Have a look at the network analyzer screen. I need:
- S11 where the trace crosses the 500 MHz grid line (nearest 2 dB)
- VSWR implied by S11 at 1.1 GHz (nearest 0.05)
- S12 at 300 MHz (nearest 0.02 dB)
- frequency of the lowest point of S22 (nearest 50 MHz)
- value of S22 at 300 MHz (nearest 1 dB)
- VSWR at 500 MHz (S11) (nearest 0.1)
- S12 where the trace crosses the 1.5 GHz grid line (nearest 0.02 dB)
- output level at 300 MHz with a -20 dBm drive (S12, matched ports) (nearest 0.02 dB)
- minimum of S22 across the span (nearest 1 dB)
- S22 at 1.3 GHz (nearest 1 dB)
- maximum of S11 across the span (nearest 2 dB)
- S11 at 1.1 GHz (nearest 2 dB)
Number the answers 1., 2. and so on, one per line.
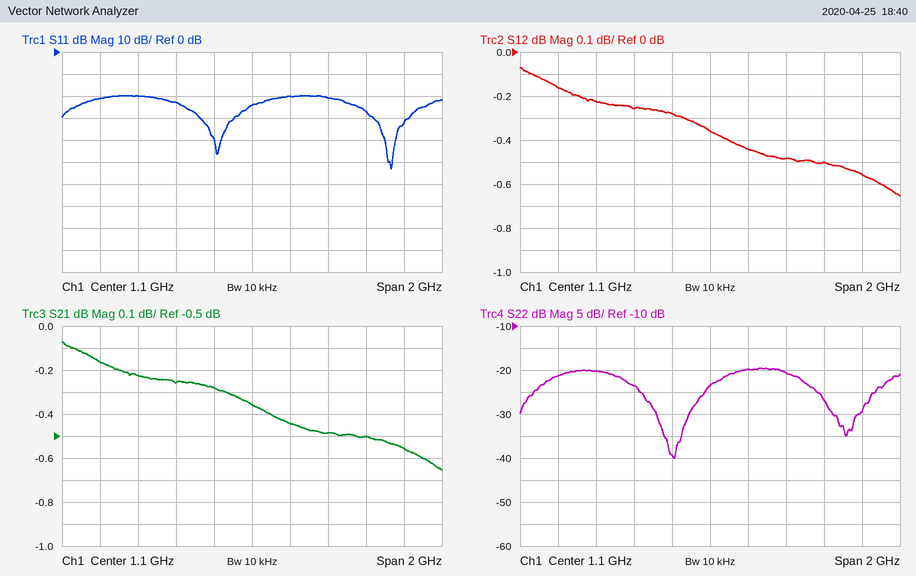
1. -20 dB
2. 1.15
3. -0.16 dB
4. 900 MHz
5. -21 dB
6. 1.2
7. -0.48 dB
8. -20.16 dBm
9. -40 dB
10. -20 dB
11. -20 dB
12. -24 dB
